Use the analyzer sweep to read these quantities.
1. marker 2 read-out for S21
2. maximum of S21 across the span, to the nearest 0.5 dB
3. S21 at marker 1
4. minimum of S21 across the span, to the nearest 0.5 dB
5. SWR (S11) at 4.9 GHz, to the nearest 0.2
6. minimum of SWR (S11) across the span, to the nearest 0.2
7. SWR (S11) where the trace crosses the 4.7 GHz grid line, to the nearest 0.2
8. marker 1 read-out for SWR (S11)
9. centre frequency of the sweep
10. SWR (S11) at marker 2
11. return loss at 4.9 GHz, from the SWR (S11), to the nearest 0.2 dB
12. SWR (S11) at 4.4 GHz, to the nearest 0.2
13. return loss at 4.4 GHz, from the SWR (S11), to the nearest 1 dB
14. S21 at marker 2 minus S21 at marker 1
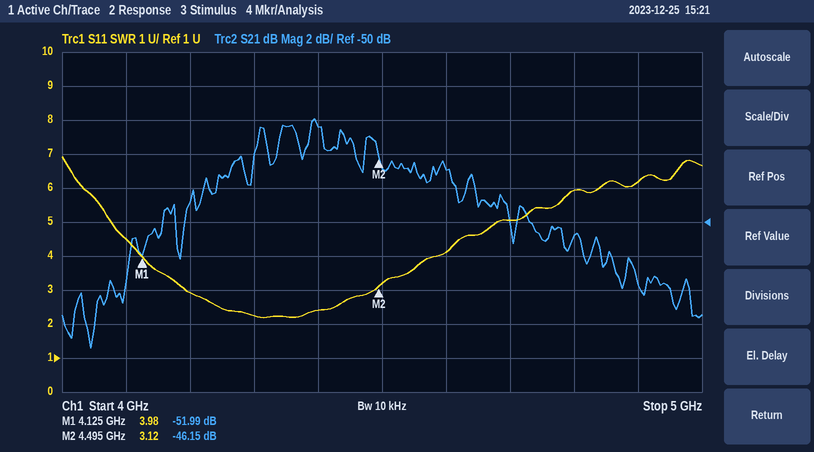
-46.15 dB
-44.0 dB
-51.99 dB
-57.5 dB
6.2
2.2
5.0
3.98
4.5 GHz
3.12
2.8 dB
2.4
8 dB
5.84 dB
